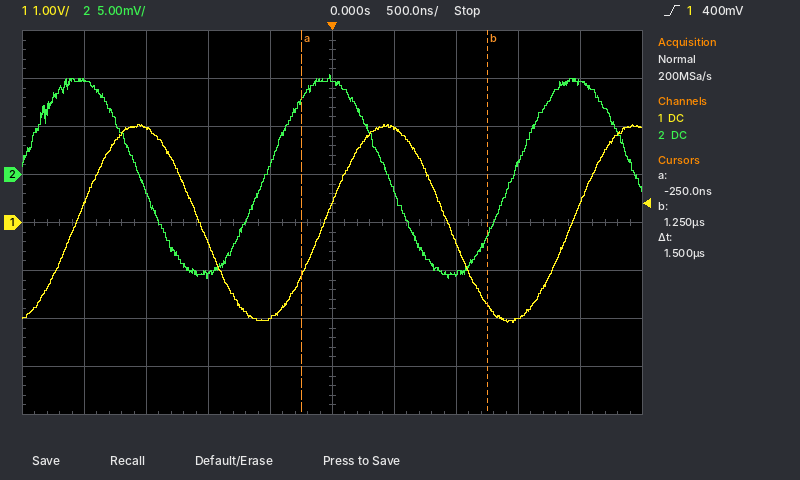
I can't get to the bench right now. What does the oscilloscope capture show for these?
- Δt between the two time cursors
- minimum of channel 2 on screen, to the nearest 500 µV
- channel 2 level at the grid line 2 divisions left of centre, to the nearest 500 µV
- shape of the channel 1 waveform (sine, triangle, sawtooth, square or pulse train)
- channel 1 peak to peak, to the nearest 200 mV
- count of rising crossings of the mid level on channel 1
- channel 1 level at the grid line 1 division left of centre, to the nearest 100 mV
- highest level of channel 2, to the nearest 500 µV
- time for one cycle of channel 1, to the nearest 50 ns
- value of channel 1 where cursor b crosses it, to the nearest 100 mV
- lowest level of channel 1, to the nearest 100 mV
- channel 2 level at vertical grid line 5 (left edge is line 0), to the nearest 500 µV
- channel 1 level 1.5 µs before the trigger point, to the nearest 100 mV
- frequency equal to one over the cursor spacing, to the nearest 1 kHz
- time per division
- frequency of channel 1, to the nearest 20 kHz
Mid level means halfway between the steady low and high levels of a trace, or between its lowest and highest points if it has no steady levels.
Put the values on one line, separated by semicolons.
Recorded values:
1.5 µs; -11.0 mV; -10.5 mV; sine; 4.2 V; 3; -2.0 V; 10.5 mV; 2.00 µs; -1.7 V; -2.1 V; 10.0 mV; 2.0 V; 667 kHz; 500 ns; 500 kHz
